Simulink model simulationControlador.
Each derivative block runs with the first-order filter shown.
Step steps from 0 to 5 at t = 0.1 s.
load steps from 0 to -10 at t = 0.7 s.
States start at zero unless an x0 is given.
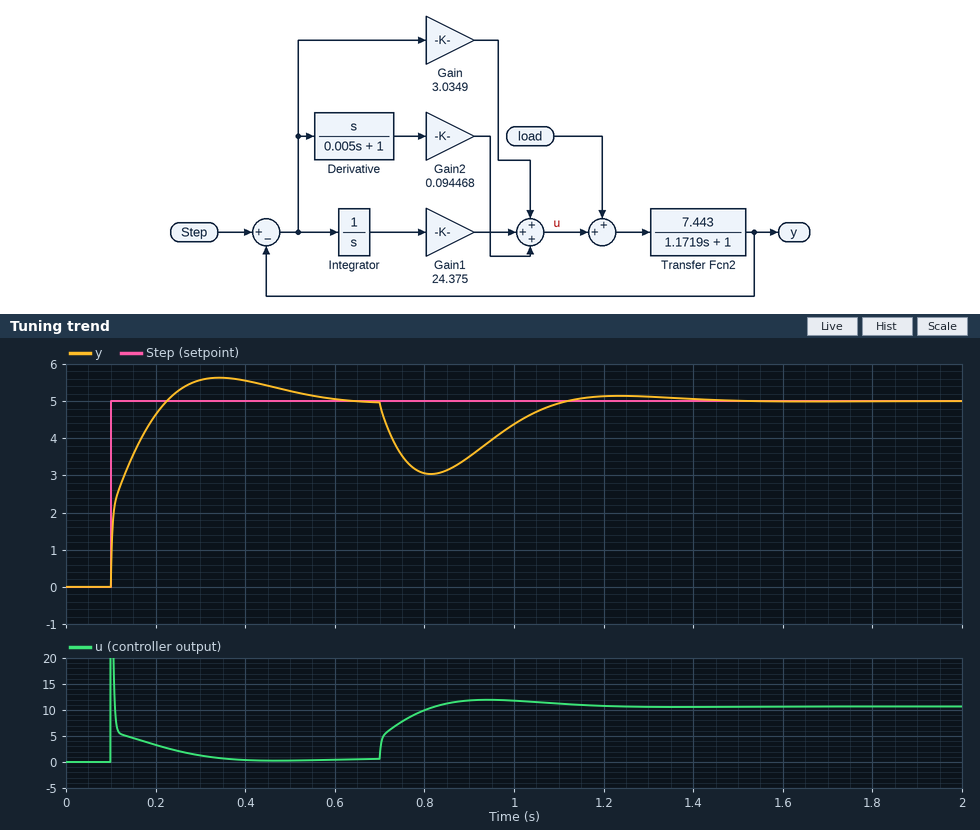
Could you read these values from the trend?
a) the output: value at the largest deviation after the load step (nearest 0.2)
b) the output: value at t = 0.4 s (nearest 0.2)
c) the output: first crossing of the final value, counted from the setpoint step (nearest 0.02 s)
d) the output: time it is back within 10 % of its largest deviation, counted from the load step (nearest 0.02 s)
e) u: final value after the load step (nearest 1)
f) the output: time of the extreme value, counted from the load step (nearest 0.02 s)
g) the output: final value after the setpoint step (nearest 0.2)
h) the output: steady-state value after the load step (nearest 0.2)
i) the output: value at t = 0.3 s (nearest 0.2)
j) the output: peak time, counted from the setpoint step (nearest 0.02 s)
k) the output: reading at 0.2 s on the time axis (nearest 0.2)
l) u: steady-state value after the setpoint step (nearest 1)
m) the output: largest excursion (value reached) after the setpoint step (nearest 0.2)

3.0
5.6
0.12 s
0.36 s
11
0.12 s
5.0
5.0
5.6
0.24 s
4.6
1
5.6
